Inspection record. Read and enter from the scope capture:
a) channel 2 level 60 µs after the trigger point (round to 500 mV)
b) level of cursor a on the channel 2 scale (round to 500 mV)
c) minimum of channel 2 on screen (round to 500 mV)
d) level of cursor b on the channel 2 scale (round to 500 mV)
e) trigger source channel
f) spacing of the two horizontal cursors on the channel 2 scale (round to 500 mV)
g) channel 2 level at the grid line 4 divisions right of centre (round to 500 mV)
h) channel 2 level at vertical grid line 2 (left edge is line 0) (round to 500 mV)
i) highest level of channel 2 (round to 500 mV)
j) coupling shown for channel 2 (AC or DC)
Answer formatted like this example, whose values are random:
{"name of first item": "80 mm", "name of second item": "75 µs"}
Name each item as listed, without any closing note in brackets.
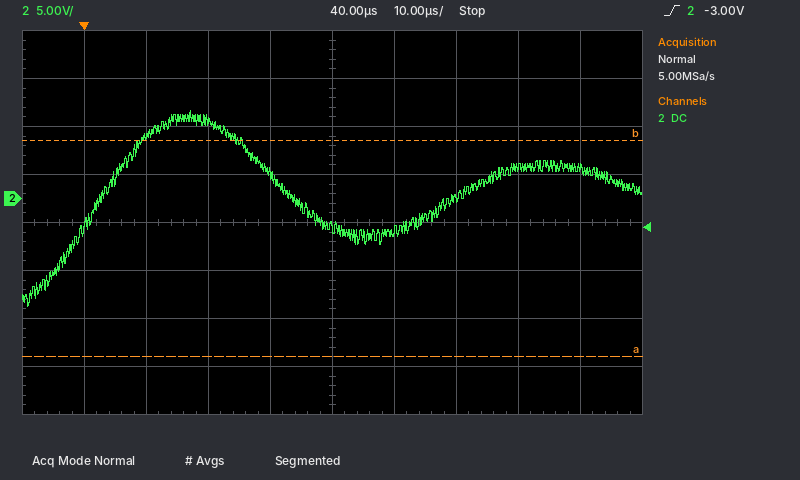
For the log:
{"channel 2 level 60 µs after the trigger point": "0.0 V", "level of cursor a on the channel 2 scale": "-16.5 V", "minimum of channel 2 on screen": "-11.0 V", "level of cursor b on the channel 2 scale": "6.0 V", "trigger source channel": "channel 2", "spacing of the two horizontal cursors on the channel 2 scale": "22.5 V", "channel 2 level at the grid line 4 divisions right of centre": "3.0 V", "channel 2 level at vertical grid line 2 (left edge is line 0)": "6.5 V", "highest level of channel 2": "9.0 V", "coupling shown for channel 2": "DC"}
